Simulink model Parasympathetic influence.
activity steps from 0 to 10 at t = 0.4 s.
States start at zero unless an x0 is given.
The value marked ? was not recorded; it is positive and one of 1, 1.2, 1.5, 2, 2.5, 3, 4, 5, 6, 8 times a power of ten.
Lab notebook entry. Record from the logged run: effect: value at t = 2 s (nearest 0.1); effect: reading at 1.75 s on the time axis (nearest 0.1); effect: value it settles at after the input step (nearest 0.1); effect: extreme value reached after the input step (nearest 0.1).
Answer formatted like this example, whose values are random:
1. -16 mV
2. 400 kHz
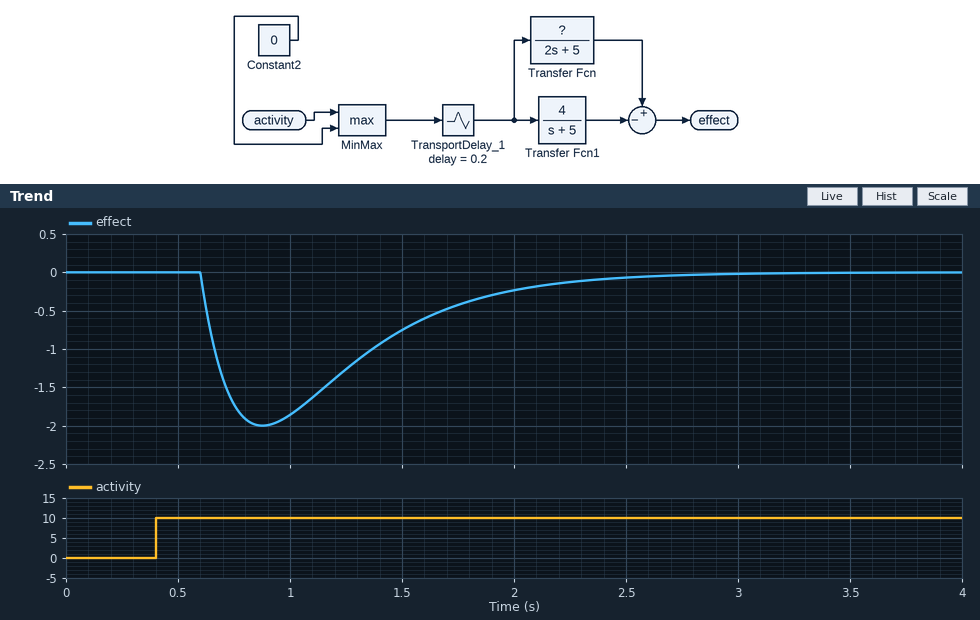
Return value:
1. -0.2
2. -0.4
3. 0.0
4. -2.0
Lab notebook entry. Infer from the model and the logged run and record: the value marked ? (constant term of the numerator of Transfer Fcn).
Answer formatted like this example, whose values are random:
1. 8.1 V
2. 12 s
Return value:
1. 4
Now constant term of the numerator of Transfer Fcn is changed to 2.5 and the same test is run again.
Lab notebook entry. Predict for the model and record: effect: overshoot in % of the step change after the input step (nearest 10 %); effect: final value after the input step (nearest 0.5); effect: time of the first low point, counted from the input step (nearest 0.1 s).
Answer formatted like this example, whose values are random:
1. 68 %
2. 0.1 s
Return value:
1. 30 %
2. -3.0
3. 0.7 s
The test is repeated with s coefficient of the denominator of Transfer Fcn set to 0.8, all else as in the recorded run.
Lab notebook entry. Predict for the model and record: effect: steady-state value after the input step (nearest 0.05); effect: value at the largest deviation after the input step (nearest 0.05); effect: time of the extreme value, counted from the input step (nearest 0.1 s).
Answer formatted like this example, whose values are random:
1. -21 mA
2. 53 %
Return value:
1. 0.00
2. 0.65
3. 0.4 s
